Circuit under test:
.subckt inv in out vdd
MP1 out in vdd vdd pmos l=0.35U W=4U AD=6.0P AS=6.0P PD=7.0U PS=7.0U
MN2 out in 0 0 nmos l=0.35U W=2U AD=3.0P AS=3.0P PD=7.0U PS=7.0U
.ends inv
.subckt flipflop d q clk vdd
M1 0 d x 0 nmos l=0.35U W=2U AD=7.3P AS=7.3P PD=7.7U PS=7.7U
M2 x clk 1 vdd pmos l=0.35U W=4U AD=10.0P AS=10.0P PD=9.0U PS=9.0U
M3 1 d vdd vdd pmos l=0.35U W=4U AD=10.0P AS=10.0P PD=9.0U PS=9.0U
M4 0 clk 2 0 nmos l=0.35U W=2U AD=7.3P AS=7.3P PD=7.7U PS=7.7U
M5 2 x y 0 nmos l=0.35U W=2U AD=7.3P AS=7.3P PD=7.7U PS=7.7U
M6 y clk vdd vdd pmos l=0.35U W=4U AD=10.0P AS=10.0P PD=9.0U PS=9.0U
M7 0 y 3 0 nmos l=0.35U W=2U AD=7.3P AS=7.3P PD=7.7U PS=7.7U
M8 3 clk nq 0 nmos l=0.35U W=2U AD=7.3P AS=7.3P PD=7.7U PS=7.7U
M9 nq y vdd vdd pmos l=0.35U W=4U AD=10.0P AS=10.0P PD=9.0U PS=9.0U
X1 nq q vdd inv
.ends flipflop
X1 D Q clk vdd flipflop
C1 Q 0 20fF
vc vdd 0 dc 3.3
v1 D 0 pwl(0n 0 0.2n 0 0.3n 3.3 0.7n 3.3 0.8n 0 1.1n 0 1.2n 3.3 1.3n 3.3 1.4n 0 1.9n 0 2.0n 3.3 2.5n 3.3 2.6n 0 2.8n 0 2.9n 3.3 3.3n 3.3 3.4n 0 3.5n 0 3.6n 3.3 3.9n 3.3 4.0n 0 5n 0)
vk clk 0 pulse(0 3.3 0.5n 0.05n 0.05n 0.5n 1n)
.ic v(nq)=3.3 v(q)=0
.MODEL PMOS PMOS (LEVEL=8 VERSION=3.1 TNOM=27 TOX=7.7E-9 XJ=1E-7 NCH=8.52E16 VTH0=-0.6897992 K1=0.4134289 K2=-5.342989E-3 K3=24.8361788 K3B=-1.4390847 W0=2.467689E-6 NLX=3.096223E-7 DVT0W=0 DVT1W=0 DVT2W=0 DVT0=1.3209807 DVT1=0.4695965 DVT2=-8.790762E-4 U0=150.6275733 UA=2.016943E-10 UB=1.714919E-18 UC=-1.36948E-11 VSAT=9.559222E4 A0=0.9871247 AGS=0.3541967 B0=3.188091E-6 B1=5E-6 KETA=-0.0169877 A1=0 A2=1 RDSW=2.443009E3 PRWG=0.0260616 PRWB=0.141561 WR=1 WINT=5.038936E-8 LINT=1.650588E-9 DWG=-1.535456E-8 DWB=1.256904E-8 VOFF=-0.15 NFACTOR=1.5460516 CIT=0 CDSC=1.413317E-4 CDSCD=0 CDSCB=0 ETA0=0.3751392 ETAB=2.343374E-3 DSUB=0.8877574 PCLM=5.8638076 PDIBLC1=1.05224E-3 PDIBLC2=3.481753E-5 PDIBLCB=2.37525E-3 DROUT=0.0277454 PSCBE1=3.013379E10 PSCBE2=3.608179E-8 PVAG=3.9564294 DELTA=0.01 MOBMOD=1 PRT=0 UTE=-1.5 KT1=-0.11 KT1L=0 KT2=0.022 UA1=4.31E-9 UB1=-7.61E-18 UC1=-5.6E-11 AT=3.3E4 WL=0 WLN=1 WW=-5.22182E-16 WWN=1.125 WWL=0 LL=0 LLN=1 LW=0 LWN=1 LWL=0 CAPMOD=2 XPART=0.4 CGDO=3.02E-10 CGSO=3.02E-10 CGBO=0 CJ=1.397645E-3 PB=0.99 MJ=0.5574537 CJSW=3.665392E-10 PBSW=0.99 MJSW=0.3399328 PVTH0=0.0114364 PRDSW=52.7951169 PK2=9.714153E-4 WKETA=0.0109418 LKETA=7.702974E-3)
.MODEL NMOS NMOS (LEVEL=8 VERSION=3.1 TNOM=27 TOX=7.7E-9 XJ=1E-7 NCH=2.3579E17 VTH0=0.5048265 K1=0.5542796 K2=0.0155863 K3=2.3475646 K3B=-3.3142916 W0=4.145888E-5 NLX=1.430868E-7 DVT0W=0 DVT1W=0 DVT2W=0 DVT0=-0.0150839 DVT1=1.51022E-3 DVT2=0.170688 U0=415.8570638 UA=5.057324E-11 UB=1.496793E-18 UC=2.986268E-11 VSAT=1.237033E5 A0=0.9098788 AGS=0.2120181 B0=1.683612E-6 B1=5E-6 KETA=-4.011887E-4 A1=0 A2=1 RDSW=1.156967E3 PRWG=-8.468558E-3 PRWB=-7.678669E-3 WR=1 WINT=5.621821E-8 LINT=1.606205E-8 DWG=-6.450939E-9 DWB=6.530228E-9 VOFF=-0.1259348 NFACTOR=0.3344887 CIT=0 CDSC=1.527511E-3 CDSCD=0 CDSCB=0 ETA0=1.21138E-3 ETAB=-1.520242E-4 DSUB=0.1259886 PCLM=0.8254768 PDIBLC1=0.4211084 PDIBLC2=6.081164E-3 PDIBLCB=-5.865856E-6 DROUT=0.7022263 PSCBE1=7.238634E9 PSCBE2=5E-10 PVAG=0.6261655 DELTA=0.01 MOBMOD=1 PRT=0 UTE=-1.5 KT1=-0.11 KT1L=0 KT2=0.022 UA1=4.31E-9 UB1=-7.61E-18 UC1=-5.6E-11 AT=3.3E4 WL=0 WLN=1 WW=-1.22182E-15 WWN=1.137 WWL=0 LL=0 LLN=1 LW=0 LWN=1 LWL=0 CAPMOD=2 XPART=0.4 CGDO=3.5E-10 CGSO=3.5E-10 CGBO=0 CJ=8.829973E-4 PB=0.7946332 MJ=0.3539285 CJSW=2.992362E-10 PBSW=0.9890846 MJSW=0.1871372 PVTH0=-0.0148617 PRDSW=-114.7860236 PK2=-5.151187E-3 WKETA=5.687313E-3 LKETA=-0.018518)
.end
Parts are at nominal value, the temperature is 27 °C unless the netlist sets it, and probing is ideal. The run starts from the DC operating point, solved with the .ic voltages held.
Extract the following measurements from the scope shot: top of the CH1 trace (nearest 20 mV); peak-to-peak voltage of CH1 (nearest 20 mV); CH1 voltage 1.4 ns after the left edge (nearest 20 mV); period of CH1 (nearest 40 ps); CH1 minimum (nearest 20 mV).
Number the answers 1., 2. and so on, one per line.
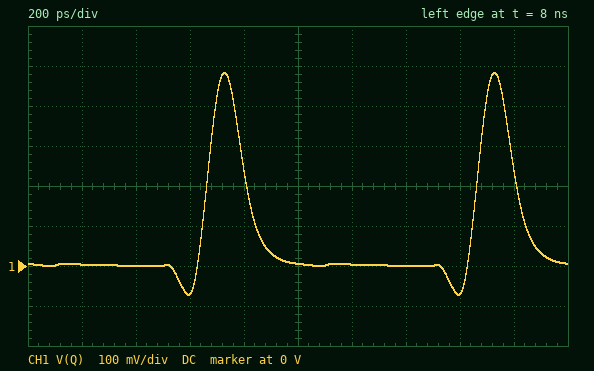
1. 480 mV
2. 560 mV
3. 0 V
4. 1.00 ns
5. -80 mV
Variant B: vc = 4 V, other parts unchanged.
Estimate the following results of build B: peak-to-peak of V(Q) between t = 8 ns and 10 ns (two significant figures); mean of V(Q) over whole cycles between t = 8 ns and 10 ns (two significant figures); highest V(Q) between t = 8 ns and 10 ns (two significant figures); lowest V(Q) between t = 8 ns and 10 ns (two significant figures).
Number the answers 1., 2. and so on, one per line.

1. 570 mV
2. 62 mV
3. 500 mV
4. -72 mV
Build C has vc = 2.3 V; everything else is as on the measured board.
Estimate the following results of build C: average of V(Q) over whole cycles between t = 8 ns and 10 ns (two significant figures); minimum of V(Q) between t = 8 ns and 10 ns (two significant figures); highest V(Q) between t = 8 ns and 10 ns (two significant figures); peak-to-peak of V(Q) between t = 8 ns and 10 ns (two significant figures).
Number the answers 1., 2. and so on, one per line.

1. 41 mV
2. -68 mV
3. 250 mV
4. 320 mV
